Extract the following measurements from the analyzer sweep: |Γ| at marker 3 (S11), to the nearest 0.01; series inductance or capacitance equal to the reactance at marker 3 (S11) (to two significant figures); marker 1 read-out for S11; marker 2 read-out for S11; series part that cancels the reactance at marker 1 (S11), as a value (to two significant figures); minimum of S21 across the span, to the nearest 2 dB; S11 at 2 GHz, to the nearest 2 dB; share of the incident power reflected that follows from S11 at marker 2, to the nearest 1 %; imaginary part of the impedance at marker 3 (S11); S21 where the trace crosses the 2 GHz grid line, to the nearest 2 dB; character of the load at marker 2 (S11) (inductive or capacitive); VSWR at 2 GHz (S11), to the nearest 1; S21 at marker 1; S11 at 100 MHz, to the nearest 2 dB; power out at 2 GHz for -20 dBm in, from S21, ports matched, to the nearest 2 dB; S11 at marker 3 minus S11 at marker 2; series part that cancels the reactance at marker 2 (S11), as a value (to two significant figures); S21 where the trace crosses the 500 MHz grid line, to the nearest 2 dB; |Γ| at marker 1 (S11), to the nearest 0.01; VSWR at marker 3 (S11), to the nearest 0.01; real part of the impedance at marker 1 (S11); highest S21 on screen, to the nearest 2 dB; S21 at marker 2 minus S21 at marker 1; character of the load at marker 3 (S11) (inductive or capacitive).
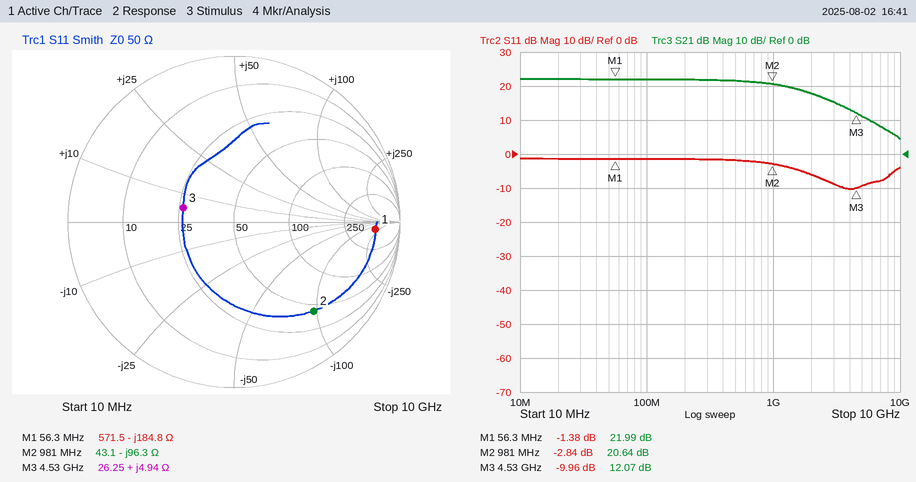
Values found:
0.32
170 pH
-1.38 dB
-2.84 dB
520 nH
4 dB
-6 dB
52 %
+4.94 Ω
18 dB
capacitive
3
21.99 dB
-2 dB
-2 dBm
-7.12 dB
16 nH
22 dB
0.85
1.93
571.5 Ω
22 dB
-1.35 dB
inductive
